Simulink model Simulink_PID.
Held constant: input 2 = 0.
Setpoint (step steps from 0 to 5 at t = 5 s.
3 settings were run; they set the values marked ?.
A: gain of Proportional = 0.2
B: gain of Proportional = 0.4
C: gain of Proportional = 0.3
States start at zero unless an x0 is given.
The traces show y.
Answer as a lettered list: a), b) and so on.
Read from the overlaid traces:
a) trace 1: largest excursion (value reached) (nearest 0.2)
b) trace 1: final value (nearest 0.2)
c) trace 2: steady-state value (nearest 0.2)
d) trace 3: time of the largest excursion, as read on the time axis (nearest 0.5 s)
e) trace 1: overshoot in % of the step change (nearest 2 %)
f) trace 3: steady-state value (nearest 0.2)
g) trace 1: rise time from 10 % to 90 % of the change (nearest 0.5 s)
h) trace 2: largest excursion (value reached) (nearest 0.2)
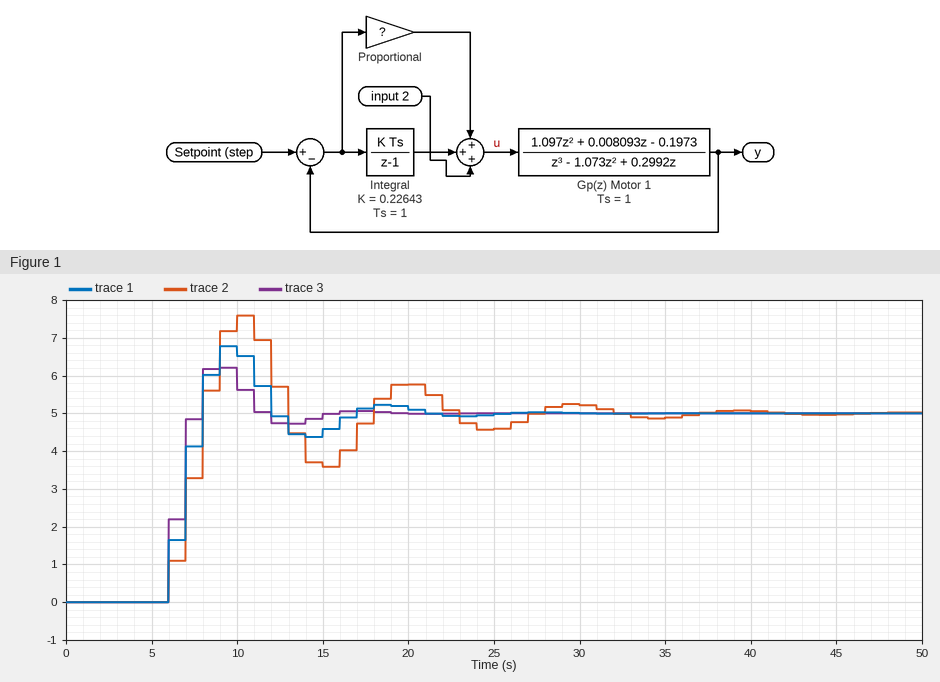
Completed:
a) 6.8
b) 5.0
c) 5.0
d) 9.0 s
e) 36 %
f) 5.0
g) 2.0 s
h) 7.6
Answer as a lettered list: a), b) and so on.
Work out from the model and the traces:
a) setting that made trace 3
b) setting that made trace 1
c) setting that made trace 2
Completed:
a) B
b) C
c) A
